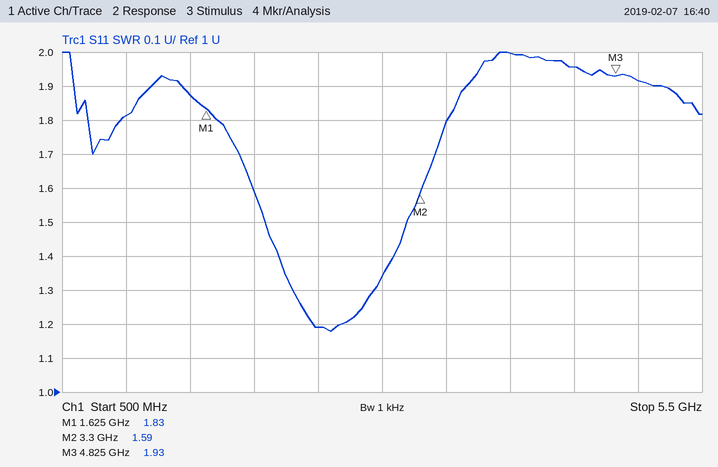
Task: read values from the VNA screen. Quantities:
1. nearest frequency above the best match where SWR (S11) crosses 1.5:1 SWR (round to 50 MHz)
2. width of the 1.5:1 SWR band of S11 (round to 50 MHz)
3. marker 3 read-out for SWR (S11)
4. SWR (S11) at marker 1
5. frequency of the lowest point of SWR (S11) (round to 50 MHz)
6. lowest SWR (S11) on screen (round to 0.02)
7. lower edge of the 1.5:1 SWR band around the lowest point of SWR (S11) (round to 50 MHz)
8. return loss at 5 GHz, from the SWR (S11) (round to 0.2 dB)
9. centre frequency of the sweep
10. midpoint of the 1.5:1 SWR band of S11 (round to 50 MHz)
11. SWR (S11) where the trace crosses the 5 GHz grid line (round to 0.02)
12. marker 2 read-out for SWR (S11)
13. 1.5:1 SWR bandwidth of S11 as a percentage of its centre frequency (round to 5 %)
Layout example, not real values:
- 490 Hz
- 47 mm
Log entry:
- 3.20 GHz
- 1.10 GHz
- 1.93
- 1.83
- 2.60 GHz
- 1.18
- 2.10 GHz
- 10.0 dB
- 3 GHz
- 2.65 GHz
- 1.92
- 1.59
- 40 %
